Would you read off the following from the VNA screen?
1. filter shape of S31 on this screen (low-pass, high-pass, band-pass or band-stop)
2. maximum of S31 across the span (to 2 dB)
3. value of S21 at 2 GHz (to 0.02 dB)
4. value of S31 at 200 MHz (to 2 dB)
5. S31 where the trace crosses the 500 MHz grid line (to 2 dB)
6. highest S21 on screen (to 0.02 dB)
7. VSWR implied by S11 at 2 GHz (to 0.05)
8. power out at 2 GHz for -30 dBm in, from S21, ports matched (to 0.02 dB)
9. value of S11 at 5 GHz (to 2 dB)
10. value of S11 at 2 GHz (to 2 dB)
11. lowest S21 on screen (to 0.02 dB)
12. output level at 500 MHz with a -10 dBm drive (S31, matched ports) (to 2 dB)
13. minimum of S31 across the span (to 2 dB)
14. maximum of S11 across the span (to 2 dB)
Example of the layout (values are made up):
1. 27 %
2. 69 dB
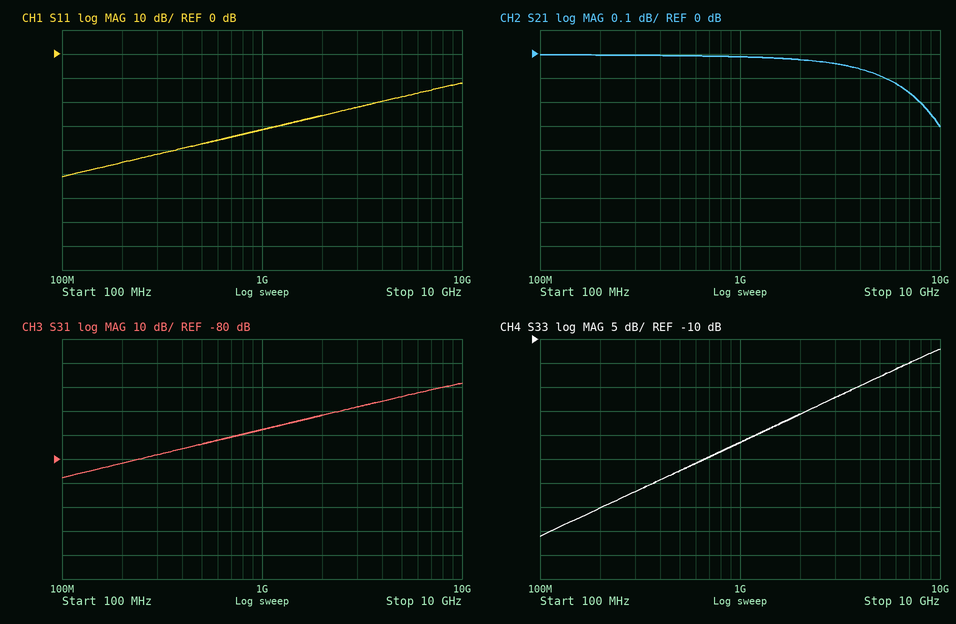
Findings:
1. high-pass
2. -48 dB
3. -0.02 dB
4. -82 dB
5. -74 dB
6. 0.00 dB
7. 1.10
8. -30.02 dBm
9. -18 dB
10. -26 dB
11. -0.30 dB
12. -84 dBm
13. -88 dB
14. -12 dB
